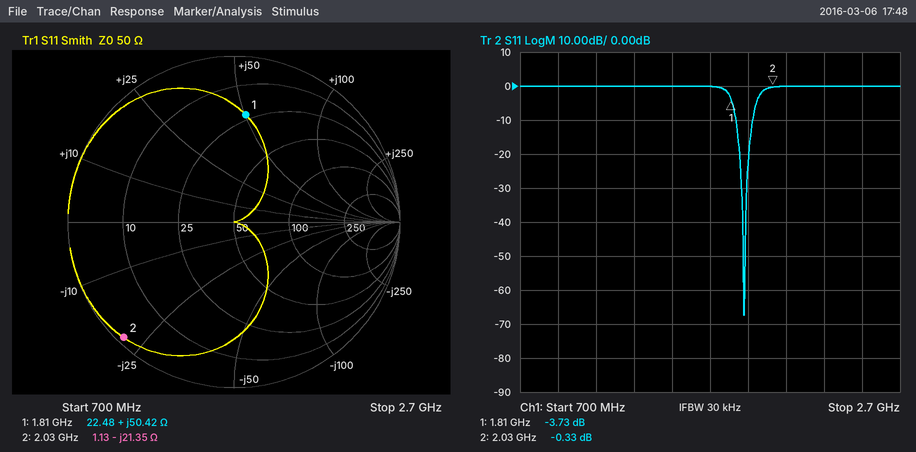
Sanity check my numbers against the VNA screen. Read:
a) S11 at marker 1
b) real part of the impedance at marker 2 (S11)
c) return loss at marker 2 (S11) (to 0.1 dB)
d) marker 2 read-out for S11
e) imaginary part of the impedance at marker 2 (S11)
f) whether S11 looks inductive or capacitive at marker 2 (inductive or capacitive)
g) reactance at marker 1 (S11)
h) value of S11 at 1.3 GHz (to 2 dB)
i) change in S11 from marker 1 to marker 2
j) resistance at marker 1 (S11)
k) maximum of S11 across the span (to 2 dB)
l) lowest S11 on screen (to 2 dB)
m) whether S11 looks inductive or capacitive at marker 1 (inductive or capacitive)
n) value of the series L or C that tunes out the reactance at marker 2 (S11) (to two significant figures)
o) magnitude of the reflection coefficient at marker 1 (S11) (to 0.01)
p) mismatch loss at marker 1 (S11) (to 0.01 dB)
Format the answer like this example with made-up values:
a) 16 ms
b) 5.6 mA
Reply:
a) -3.73 dB
b) 1.13 Ω
c) 0.3 dB
d) -0.33 dB
e) -21.35 Ω
f) capacitive
g) +50.42 Ω
h) 0 dB
i) 3.40 dB
j) 22.48 Ω
k) 0 dB
l) -68 dB
m) inductive
n) 1.7 nH
o) 0.65
p) 2.39 dB
